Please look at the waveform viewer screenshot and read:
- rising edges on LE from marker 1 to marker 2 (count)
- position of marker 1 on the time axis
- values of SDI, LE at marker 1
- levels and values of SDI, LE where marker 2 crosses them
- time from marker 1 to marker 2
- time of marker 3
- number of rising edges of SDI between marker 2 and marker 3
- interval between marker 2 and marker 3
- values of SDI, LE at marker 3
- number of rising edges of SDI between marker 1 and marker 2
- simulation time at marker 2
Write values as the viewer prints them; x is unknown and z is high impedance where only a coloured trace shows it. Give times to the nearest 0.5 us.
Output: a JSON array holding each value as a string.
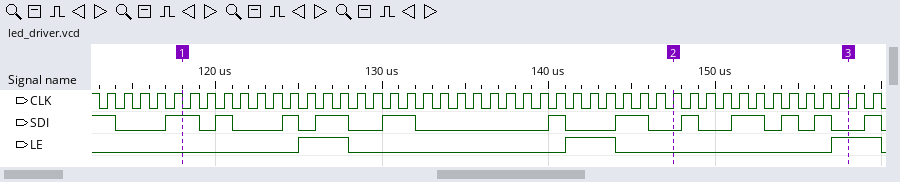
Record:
["2", "118 us", "SDI=1, LE=0", "SDI=0, LE=0", "29.5 us", "158 us", "4", "10.5 us", "SDI=0, LE=1", "6", "147.5 us"]
